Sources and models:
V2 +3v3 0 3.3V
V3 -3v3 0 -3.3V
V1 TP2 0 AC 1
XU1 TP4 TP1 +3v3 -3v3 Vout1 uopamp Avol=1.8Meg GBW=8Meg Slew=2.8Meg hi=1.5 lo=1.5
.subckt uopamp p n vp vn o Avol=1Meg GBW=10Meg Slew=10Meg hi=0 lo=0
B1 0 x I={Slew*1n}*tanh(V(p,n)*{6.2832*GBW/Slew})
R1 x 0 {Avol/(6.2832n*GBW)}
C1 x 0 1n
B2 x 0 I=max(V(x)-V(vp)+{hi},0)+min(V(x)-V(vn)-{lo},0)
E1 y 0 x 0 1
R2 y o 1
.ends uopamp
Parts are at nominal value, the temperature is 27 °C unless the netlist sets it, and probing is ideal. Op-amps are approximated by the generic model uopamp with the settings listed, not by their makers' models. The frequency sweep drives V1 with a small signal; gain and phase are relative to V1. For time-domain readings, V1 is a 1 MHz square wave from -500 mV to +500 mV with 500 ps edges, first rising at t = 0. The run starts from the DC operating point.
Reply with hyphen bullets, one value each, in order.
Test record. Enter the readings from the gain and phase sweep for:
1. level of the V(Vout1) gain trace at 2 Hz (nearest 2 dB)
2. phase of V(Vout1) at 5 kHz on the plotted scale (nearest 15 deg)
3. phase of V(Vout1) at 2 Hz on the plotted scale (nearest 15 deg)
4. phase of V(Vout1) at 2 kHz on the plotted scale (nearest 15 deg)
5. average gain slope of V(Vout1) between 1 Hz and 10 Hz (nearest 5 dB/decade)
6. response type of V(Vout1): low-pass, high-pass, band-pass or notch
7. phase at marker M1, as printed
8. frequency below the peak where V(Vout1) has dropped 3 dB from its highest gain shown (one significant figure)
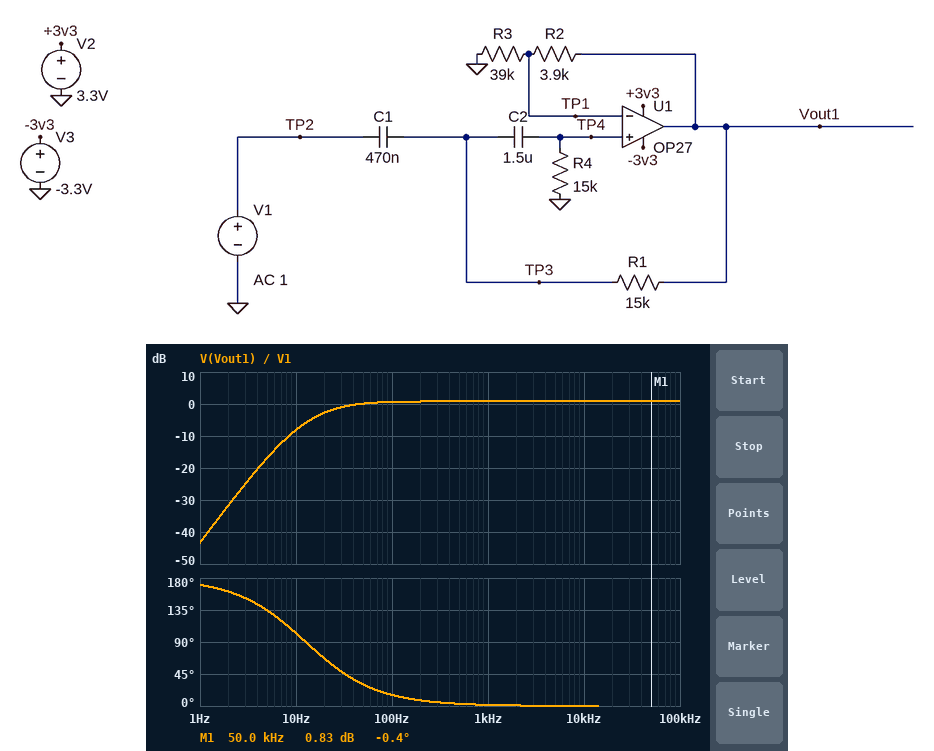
- -32 dB
- 0 deg
- 165 deg
- 0 deg
- 35 dB/decade
- high-pass
- -0.4 deg
- 20 Hz
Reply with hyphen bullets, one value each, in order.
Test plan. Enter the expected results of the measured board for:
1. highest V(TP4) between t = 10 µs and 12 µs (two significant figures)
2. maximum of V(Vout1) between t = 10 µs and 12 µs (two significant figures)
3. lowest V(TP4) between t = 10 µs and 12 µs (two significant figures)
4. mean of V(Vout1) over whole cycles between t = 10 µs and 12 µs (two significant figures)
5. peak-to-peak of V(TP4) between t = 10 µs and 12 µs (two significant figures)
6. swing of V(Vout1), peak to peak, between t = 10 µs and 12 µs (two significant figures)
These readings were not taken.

- 1.0 V
- 1.1 V
- -1.1 mV
- 550 mV
- 1.0 V
- 1.1 V
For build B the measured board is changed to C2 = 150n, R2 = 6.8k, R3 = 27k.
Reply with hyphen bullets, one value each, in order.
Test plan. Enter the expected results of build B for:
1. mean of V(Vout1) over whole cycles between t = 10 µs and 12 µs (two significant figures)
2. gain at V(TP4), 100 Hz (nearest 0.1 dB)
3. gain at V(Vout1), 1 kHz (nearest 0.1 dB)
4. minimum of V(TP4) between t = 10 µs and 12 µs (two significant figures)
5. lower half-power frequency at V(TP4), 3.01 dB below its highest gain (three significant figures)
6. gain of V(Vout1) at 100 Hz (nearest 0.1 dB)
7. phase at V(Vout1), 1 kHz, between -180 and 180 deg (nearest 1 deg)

- 620 mV
- -1.7 dB
- 1.9 dB
- -3.3 mV
- 70.7 Hz
- 0.3 dB
- 5 deg
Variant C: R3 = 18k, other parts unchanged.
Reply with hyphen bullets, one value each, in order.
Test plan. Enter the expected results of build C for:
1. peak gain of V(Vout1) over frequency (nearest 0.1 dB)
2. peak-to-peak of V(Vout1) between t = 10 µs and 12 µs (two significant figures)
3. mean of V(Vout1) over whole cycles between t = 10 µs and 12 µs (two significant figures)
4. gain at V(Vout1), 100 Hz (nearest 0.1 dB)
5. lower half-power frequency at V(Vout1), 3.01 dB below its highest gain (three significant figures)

- 1.7 dB
- 1.2 V
- 610 mV
- 1.6 dB
- 19.1 Hz
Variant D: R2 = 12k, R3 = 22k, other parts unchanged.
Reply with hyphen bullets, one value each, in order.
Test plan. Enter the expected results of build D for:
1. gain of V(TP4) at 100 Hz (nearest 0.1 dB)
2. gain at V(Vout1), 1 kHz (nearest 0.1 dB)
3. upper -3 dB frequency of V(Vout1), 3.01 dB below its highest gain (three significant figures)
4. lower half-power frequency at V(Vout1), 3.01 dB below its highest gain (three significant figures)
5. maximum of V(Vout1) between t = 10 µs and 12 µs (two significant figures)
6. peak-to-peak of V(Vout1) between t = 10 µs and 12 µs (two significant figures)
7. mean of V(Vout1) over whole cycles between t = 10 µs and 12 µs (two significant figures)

- 0 dB
- 3.8 dB
- 5.16 MHz
- 12.3 Hz
- 1.5 V
- 1.4 V
- 770 mV
